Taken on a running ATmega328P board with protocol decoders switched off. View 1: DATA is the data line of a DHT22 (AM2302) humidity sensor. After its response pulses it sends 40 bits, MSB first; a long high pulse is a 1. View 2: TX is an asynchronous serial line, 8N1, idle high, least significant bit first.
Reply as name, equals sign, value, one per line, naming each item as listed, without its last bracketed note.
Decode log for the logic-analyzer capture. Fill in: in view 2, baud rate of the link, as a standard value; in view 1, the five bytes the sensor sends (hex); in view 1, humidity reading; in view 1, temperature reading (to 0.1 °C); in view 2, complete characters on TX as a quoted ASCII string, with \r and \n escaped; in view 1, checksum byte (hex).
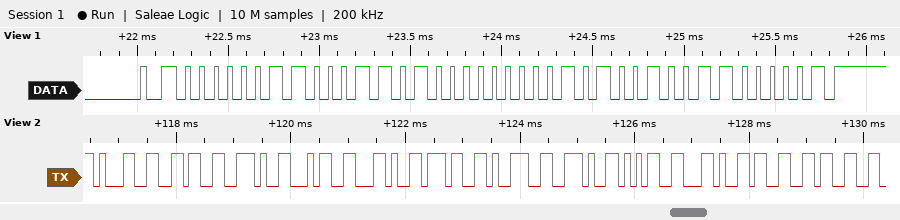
in view 2, baud rate of the link, as a standard value = 9600 baud
in view 1, the five bytes the sensor sends = 03 1A 00 A4 C1
in view 1, humidity reading = 79.4 %
in view 1, temperature reading = 16.4 °C
in view 2, complete characters on TX as a quoted ASCII string, with \r and \n escaped = "16.4,79.5,33"
in view 1, checksum byte = 0xC1
